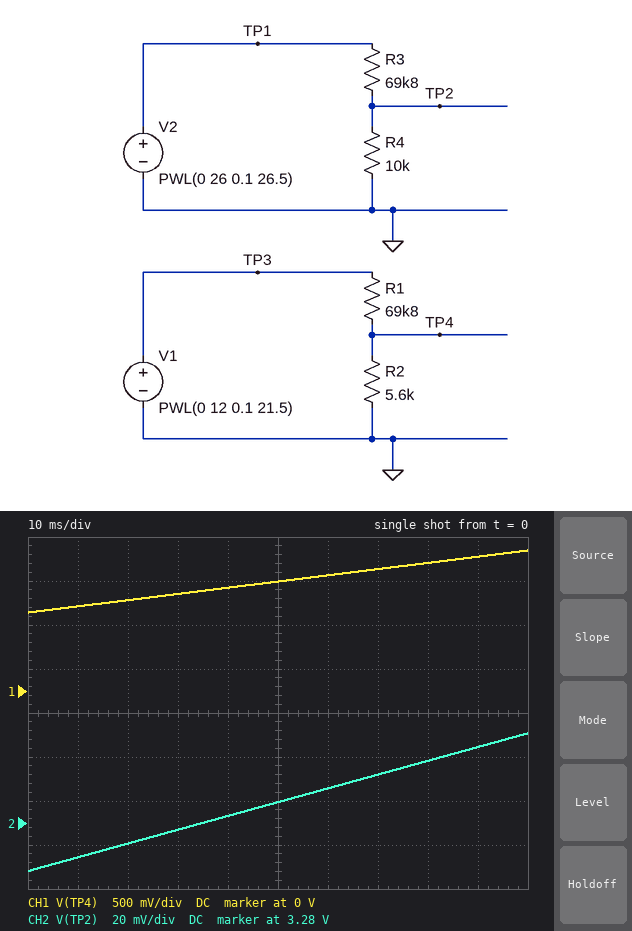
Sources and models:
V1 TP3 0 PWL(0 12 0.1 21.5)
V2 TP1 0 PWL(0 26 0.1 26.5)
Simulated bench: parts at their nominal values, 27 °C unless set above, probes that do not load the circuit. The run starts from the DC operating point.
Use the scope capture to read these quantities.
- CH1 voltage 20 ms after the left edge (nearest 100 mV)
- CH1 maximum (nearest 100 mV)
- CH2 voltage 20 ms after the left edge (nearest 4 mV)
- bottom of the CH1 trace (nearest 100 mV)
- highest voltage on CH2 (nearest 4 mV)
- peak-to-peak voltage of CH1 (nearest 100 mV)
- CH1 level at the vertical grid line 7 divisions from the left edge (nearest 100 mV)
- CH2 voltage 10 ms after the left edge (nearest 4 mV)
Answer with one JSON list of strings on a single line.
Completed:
["1.0 V", "1.6 V", "3.272 V", "900 mV", "3.320 V", "700 mV", "1.4 V", "3.264 V"]
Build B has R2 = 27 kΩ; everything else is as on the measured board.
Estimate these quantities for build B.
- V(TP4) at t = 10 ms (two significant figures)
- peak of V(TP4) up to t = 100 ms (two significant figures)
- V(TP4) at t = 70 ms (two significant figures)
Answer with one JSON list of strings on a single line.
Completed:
["3.6 V", "6.0 V", "5.2 V"]
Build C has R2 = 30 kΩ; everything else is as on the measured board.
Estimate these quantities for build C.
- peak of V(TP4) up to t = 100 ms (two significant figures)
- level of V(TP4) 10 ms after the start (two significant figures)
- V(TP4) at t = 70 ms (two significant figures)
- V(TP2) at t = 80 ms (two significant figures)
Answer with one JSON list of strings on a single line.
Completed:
["6.5 V", "3.9 V", "5.6 V", "3.3 V"]
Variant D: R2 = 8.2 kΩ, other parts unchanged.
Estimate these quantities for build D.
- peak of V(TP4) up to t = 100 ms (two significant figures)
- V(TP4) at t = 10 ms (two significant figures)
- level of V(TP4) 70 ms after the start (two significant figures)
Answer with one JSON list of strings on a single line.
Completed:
["2.3 V", "1.4 V", "2.0 V"]
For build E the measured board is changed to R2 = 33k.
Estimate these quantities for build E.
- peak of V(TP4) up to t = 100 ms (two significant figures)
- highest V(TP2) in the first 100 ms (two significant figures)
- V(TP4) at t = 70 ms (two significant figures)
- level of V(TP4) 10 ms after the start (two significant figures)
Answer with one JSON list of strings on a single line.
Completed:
["6.9 V", "3.3 V", "6.0 V", "4.2 V"]
